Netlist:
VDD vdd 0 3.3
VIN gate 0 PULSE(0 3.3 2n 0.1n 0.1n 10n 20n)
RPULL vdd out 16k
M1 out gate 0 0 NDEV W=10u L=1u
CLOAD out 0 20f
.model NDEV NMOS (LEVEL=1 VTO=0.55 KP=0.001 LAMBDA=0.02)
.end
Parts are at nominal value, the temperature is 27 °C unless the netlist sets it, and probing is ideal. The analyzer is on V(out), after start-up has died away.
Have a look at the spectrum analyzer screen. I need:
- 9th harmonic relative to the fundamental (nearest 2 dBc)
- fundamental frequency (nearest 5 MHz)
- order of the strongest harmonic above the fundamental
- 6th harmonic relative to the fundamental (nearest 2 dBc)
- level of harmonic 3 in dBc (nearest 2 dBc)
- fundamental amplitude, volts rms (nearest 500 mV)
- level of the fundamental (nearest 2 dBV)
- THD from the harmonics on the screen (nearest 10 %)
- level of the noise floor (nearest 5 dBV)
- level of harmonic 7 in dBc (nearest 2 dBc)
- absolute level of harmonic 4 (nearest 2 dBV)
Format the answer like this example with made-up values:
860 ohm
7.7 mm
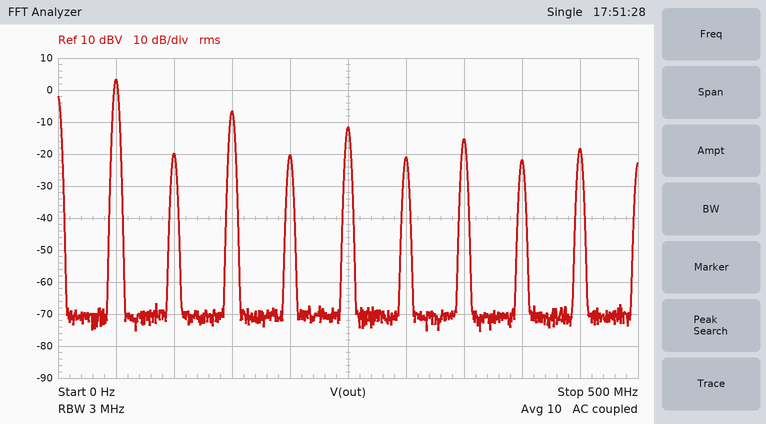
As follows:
-22 dBc
50 MHz
3
-24 dBc
-10 dBc
1.5 V
4 dBV
40 %
-70 dBV
-18 dBc
-20 dBV
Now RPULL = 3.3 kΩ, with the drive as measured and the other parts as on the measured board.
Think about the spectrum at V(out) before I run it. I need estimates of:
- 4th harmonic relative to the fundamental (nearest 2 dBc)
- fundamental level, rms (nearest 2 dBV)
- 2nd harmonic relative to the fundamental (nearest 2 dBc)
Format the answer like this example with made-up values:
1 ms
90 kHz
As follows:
-30 dBc
4 dBV
-30 dBc
